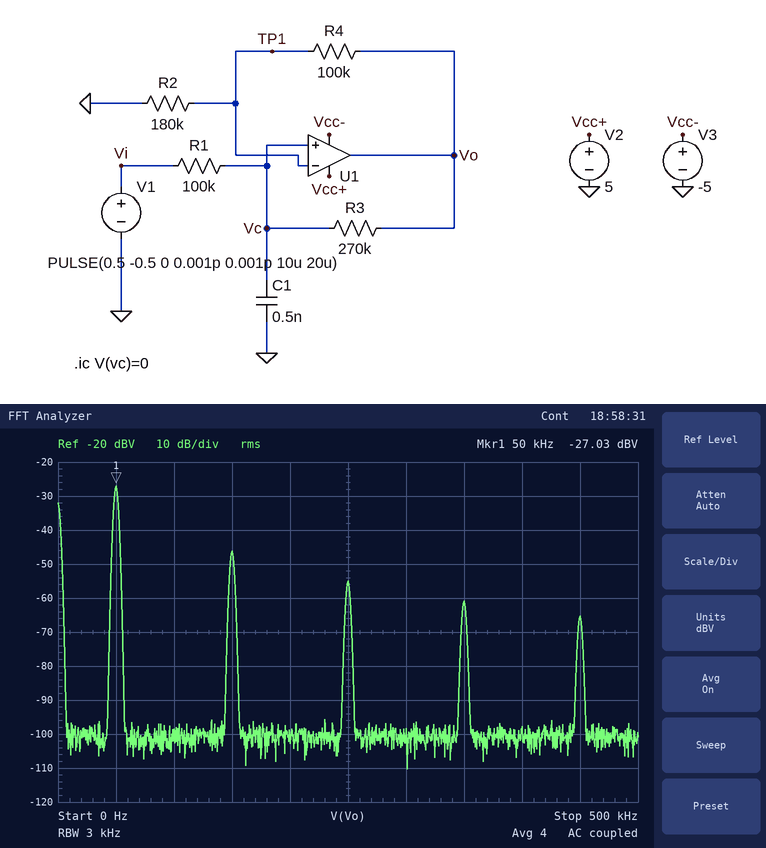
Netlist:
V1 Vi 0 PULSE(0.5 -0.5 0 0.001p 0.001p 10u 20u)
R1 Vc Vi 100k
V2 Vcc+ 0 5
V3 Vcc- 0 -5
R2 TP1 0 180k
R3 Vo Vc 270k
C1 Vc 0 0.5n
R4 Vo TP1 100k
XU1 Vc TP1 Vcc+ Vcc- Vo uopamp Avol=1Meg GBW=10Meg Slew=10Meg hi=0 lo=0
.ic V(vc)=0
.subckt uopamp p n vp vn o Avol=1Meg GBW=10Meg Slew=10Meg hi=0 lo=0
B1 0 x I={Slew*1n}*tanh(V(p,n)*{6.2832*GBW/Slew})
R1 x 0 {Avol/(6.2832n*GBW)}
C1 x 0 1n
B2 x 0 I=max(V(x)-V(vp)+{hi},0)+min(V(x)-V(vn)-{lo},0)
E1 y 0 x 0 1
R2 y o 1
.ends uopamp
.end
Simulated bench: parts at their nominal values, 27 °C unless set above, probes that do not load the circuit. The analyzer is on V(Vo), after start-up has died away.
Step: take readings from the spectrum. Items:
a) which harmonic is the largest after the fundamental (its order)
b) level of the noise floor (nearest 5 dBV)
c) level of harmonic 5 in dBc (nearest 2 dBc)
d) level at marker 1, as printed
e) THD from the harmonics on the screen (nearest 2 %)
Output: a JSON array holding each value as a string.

["3", "-100 dBV", "-28 dBc", "-27.03 dBV", "12 %"]
